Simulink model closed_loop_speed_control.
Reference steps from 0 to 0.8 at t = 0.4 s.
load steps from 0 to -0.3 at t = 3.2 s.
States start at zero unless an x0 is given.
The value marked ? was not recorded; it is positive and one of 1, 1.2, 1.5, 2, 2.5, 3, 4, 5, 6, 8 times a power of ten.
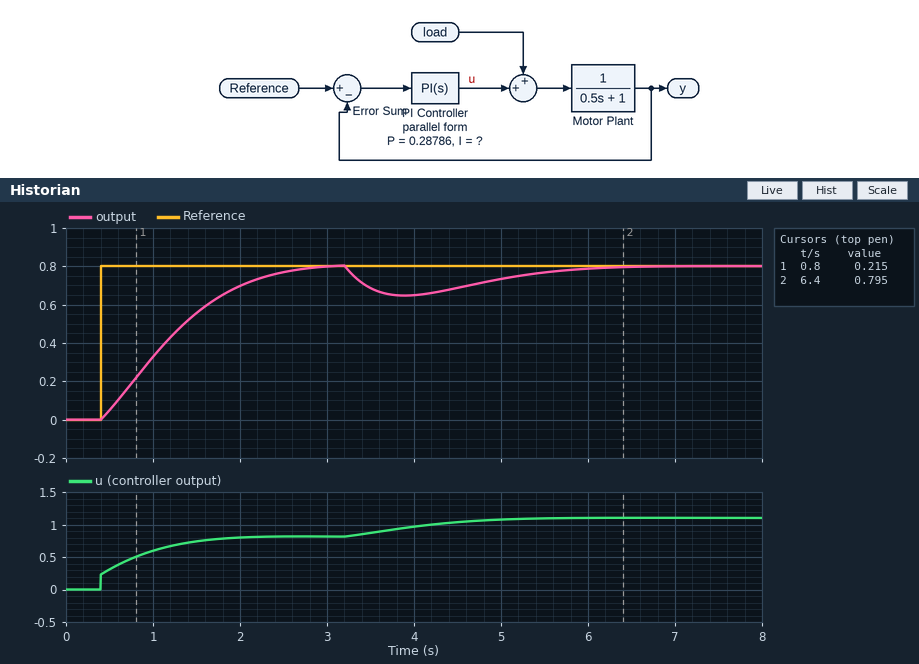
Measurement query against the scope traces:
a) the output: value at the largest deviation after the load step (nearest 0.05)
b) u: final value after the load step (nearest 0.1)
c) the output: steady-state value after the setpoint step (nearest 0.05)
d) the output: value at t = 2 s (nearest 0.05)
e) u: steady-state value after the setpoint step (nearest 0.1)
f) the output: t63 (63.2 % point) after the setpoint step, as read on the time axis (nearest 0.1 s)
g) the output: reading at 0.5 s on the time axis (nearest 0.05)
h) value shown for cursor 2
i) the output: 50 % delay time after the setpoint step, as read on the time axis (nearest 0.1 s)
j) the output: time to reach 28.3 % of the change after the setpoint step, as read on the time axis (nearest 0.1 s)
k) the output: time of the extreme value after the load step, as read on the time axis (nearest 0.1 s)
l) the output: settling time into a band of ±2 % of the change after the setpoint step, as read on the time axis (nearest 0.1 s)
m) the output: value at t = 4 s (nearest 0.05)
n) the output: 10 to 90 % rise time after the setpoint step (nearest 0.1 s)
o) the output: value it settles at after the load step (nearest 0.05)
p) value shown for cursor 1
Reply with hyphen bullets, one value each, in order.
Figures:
- 0.65
- 1.1
- 0.80
- 0.70
- 0.8
- 1.4 s
- 0.05
- 0.795
- 1.1 s
- 0.8 s
- 3.9 s
- 2.7 s
- 0.65
- 1.6 s
- 0.80
- 0.215
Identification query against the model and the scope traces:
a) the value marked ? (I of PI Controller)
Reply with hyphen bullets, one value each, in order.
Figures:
- 1.2
